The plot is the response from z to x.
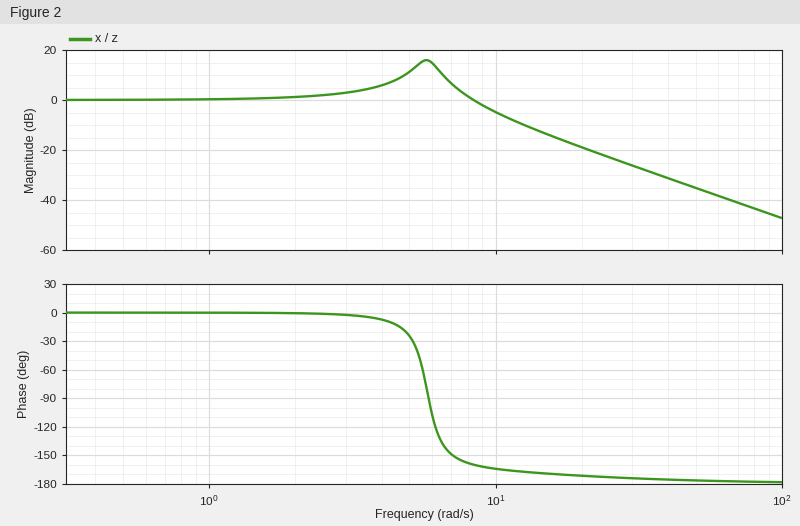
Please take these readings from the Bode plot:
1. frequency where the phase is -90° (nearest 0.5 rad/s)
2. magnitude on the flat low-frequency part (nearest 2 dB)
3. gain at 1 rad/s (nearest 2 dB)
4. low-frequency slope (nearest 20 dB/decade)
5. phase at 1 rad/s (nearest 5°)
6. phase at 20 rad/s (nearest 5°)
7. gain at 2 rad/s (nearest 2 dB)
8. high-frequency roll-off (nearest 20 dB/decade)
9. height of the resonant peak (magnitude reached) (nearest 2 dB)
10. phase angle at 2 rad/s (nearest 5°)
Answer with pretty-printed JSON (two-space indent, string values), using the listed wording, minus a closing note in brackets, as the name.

{
  "frequency where the phase is -90°": "6.0 rad/s",
  "magnitude on the flat low-frequency part": "0 dB",
  "gain at 1 rad/s": "0 dB",
  "low-frequency slope": "0 dB/decade",
  "phase at 1 rad/s": "0°",
  "phase at 20 rad/s": "-170°",
  "gain at 2 rad/s": "2 dB",
  "high-frequency roll-off": "-40 dB/decade",
  "height of the resonant peak (magnitude reached)": "16 dB",
  "phase angle at 2 rad/s": "0°"
}
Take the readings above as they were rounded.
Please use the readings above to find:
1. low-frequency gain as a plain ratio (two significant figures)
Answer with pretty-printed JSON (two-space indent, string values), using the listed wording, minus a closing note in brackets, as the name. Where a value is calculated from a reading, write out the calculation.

{
  "low-frequency gain as a plain ratio": "10^(0 / 20) = 1.0"
}
